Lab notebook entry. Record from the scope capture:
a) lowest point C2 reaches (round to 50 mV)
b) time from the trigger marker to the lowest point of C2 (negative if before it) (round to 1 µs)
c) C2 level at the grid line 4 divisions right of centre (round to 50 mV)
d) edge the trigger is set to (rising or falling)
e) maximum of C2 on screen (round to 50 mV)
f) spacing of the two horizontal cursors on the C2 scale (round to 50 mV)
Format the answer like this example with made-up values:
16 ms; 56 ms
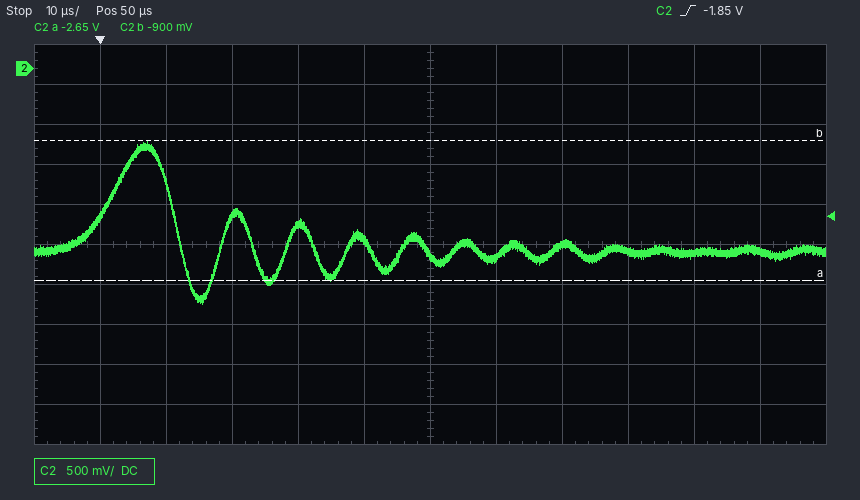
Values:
-2.95 V; +15 µs; -2.30 V; rising; -900 mV; 1.75 V
